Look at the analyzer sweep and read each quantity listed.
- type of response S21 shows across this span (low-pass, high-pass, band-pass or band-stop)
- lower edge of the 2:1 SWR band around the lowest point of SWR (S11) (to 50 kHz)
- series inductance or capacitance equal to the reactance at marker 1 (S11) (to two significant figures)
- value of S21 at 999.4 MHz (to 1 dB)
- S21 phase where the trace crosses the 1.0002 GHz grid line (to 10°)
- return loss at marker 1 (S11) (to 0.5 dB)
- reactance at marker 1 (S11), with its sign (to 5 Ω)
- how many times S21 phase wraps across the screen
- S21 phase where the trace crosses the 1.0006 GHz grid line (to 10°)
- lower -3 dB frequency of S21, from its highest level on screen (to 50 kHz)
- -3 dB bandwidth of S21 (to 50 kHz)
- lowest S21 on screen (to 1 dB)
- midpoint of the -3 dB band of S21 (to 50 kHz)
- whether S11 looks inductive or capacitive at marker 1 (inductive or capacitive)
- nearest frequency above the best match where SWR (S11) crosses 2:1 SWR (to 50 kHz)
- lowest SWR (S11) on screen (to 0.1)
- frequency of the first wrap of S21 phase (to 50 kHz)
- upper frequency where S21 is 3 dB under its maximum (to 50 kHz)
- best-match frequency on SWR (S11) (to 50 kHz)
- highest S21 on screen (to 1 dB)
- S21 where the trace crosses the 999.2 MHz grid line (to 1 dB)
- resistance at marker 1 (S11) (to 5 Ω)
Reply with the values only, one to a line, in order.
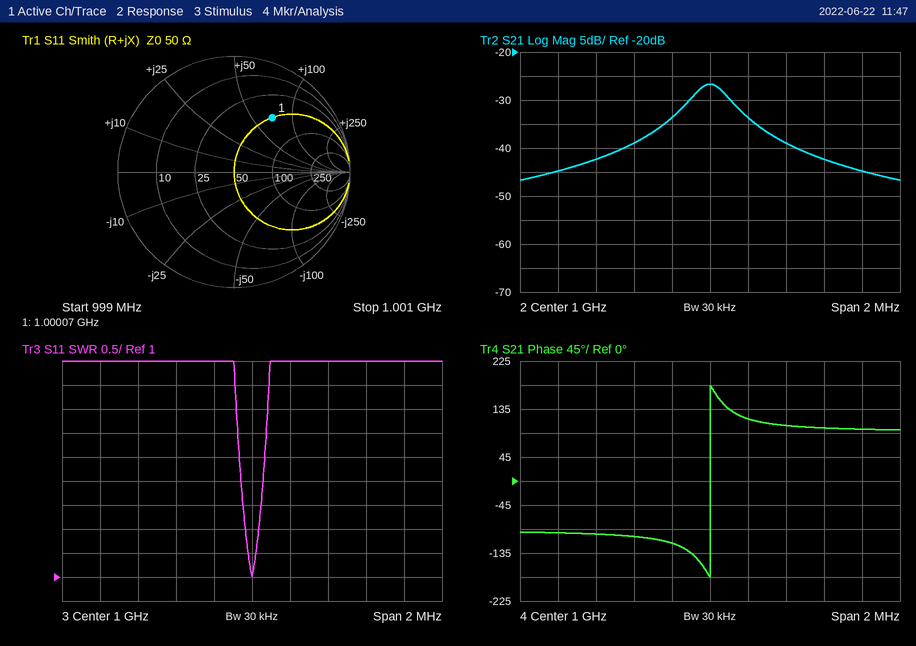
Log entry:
band-pass
999.95 MHz
11 nH
-42 dB
120°
5.0 dB
+70 Ω
1
100°
999.90 MHz
200 kHz
-47 dB
1.00000 GHz
inductive
1.00005 GHz
1.0
1.00000 GHz
1.00010 GHz
1.00000 GHz
-27 dB
-45 dB
50 Ω
